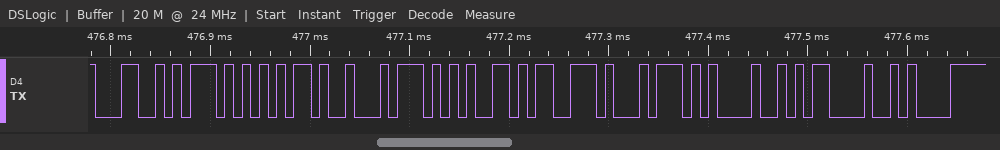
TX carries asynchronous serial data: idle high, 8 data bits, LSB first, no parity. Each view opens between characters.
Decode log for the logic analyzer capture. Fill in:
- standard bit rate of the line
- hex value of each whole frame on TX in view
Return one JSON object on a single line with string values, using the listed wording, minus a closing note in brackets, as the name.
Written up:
{"standard bit rate of the line": "115200 baud", "hex value of each whole frame on TX in view": "4C, 57, 2D, 74, 65, 73, 74, 21, 0D, 0A"}
